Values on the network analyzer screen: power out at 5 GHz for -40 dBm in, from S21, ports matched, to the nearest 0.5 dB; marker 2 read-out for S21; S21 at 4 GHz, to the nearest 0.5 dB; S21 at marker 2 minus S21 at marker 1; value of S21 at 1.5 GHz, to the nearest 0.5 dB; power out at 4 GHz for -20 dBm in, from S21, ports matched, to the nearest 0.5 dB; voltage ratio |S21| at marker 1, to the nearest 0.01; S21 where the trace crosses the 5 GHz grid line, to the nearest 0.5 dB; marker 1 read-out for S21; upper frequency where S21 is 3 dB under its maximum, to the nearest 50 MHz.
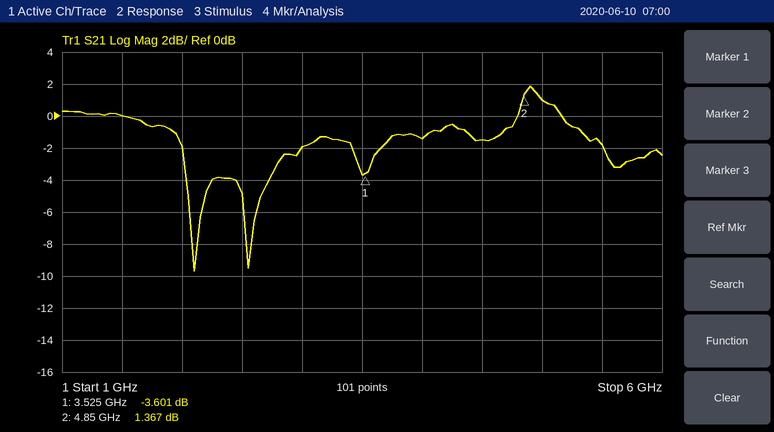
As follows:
-39.0 dBm
1.367 dB
-1.5 dB
4.968 dB
0.0 dB
-21.5 dBm
0.66
1.0 dB
-3.601 dB
5.35 GHz
